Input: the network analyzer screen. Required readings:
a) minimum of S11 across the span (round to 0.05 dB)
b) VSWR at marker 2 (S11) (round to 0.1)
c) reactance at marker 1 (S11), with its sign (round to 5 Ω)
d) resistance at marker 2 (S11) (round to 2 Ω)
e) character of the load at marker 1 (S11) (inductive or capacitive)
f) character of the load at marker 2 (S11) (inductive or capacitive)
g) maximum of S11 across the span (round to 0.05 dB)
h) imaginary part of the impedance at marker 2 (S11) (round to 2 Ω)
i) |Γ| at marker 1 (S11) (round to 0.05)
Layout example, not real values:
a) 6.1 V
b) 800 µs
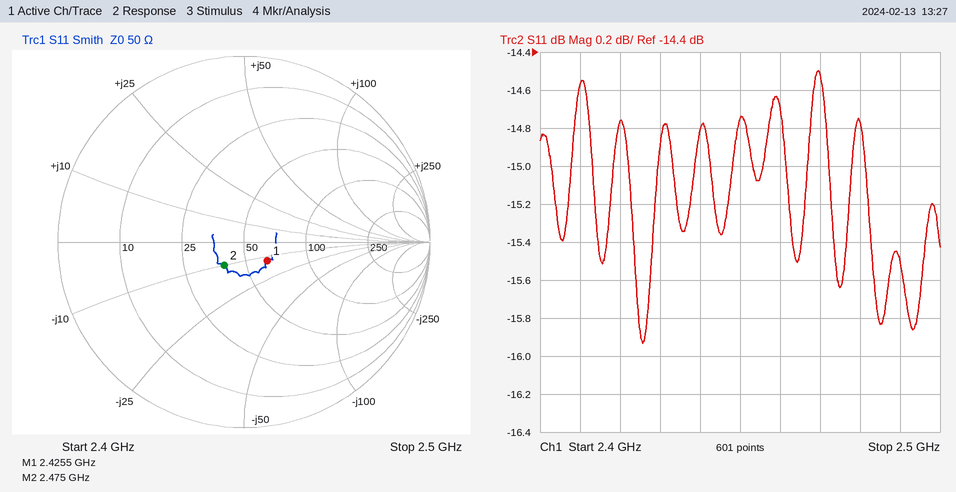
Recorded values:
a) -15.95 dB
b) 1.4
c) -15 Ω
d) 40 Ω
e) capacitive
f) capacitive
g) -14.50 dB
h) -10 Ω
i) 0.15
